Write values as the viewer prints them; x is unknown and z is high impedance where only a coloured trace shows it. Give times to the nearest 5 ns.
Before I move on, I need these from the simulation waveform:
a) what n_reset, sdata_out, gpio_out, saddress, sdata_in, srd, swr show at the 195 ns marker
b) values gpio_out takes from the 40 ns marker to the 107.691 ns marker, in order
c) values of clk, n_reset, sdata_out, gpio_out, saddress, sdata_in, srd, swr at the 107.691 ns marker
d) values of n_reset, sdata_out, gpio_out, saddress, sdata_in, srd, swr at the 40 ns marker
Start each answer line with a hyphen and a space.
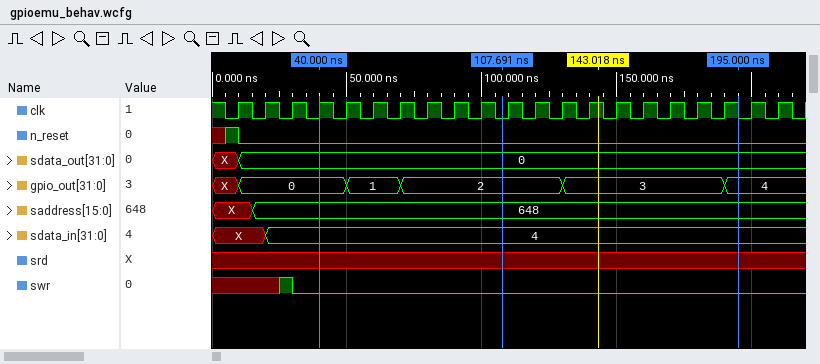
- n_reset=0, sdata_out=0, gpio_out=4, saddress=648, sdata_in=4, srd=x, swr=0
- 0, 1, 2
- clk=0, n_reset=0, sdata_out=0, gpio_out=2, saddress=648, sdata_in=4, srd=x, swr=0
- n_reset=0, sdata_out=0, gpio_out=0, saddress=648, sdata_in=4, srd=x, swr=0
